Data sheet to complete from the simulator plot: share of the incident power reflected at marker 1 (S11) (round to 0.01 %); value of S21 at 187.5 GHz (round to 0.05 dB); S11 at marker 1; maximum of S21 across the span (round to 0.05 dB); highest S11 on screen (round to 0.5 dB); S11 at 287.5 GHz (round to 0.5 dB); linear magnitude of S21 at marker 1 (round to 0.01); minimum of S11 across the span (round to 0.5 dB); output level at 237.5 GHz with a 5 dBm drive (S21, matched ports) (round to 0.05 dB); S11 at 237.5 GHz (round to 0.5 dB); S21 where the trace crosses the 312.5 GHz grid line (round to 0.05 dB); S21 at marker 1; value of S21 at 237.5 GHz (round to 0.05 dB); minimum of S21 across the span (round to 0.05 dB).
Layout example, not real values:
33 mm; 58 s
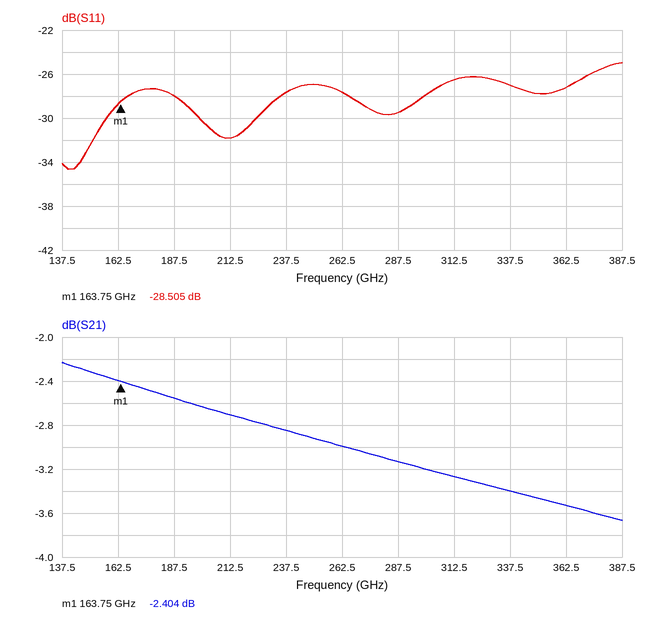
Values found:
0.14 %; -2.55 dB; -28.505 dB; -2.25 dB; -25.0 dB; -29.5 dB; 0.76; -34.5 dB; 2.15 dBm; -27.5 dB; -3.25 dB; -2.404 dB; -2.85 dB; -3.65 dB
